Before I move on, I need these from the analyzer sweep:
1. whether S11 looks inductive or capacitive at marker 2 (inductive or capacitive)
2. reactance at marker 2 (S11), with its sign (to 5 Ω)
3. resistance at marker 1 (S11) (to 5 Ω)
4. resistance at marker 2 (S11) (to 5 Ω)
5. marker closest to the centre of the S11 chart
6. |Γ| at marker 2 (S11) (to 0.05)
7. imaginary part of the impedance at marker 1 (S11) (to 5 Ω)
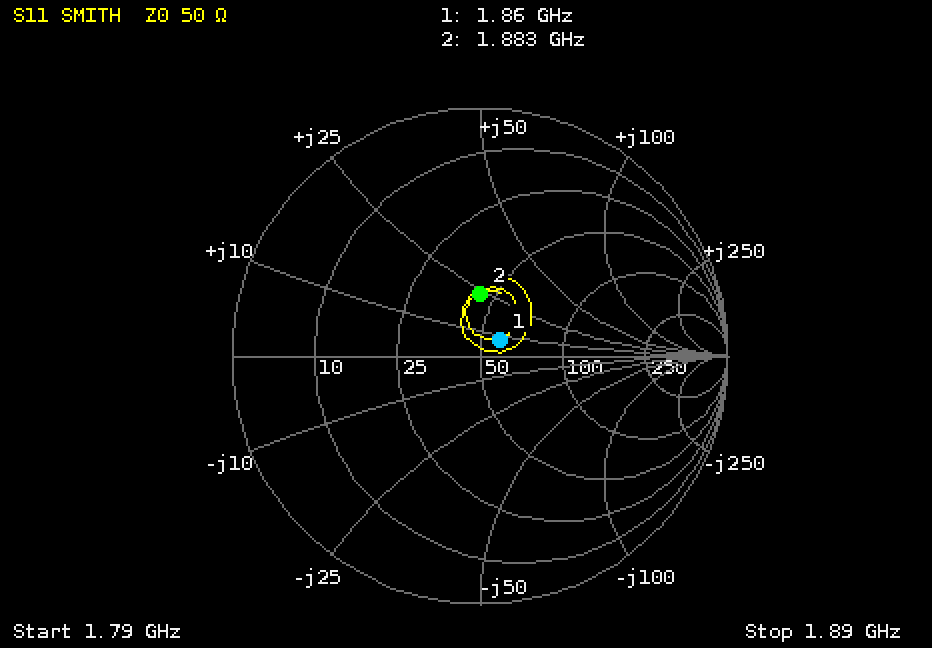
inductive
+25 Ω
60 Ω
45 Ω
marker 1
0.25
+10 Ω
